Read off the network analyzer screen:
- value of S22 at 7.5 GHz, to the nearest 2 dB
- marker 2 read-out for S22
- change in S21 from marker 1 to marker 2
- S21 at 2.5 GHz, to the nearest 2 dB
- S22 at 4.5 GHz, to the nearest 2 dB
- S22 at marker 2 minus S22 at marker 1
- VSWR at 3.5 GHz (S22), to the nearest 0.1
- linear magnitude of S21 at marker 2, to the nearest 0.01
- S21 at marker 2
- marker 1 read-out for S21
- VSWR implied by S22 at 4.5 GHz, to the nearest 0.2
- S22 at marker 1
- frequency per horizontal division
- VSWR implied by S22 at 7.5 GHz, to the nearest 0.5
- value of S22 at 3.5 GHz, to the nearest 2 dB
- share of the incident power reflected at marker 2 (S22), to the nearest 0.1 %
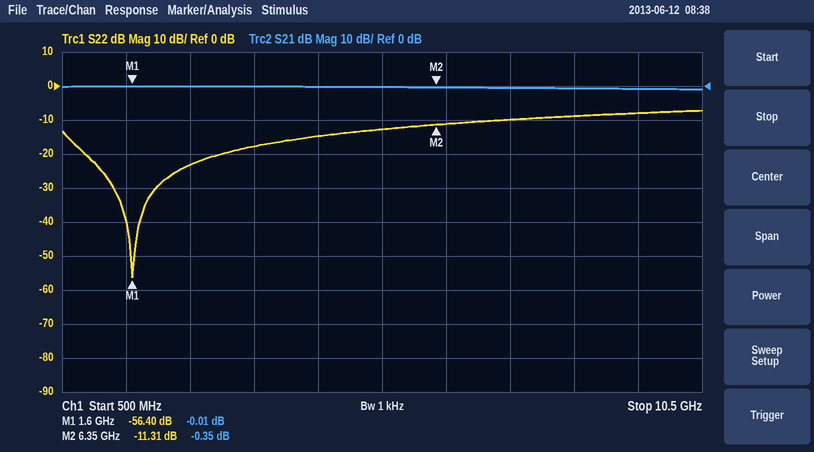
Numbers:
-10 dB
-11.31 dB
-0.34 dB
0 dB
-14 dB
45.09 dB
1.3
0.96
-0.35 dB
-0.01 dB
1.4
-56.40 dB
1 GHz
2.0
-18 dB
7.4 %
